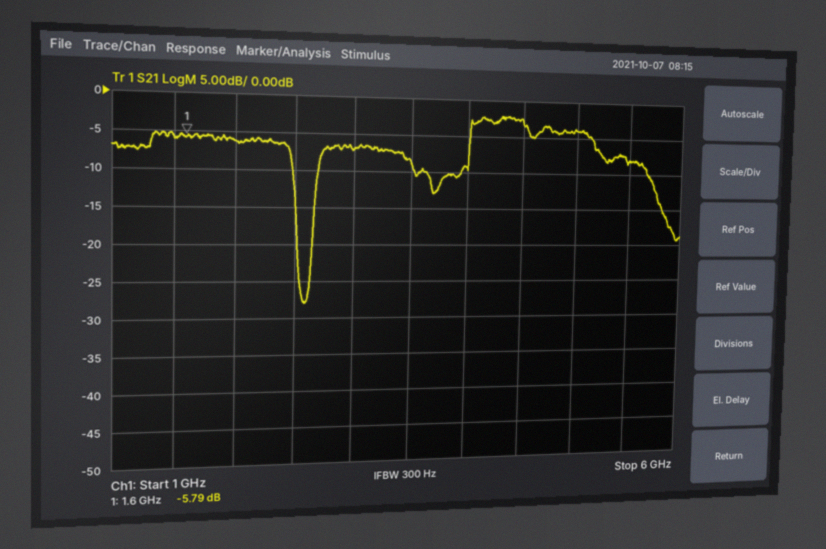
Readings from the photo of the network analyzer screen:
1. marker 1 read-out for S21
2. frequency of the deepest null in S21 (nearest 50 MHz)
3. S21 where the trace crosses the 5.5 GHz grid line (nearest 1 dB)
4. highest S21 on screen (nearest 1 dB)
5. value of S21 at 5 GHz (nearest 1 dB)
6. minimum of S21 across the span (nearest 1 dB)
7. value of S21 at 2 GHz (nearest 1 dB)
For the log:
-5.79 dB
2.60 GHz
-8 dB
-2 dB
-4 dB
-28 dB
-6 dB
